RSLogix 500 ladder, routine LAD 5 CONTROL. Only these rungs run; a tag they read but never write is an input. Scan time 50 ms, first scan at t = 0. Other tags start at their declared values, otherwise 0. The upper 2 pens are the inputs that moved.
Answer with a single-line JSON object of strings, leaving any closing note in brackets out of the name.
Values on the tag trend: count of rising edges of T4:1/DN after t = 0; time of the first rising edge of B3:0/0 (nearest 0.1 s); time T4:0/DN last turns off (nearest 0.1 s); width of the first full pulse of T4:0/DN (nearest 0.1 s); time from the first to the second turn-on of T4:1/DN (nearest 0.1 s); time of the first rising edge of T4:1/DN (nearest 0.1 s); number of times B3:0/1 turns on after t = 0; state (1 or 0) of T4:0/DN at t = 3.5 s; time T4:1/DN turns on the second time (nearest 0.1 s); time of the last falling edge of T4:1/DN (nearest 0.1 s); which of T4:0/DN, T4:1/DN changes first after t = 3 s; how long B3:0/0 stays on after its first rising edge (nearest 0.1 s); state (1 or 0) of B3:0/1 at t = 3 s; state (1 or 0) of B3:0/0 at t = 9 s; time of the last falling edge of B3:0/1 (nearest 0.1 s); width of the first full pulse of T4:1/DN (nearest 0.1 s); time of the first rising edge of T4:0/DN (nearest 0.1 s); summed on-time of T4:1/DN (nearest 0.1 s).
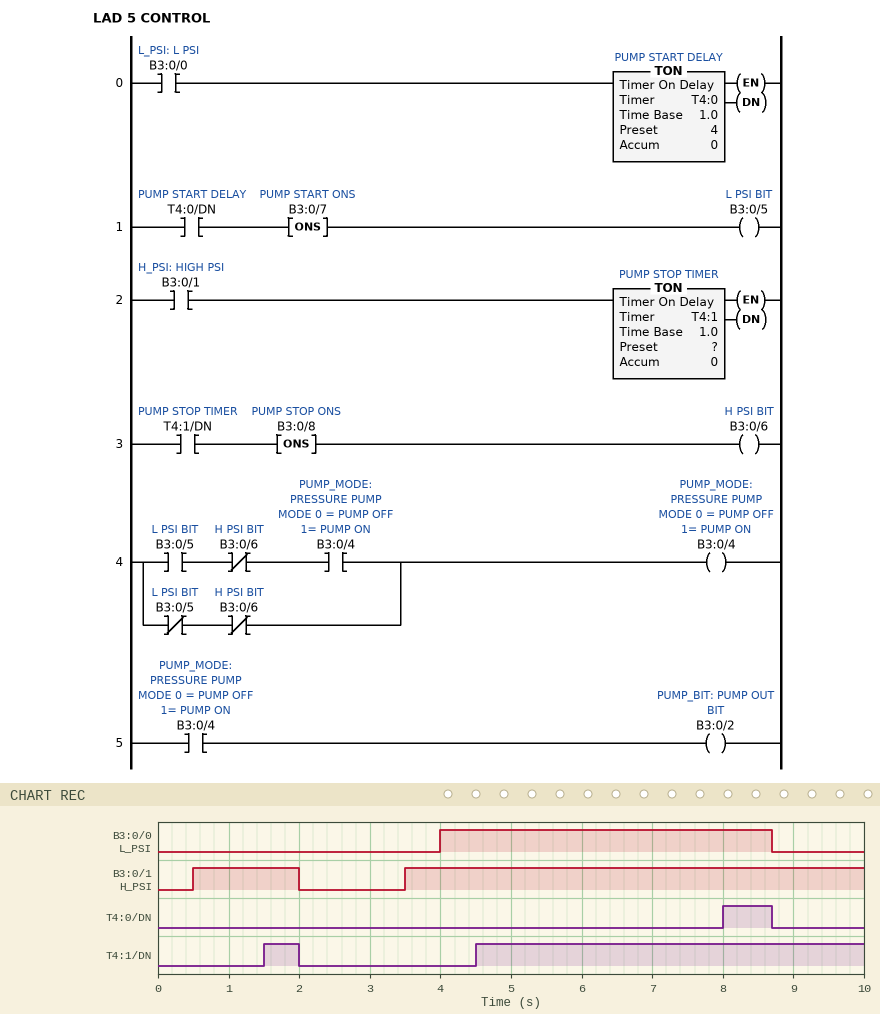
{"count of rising edges of T4:1/DN after t = 0": "2", "time of the first rising edge of B3:0/0": "4.0 s", "time T4:0/DN last turns off": "8.7 s", "width of the first full pulse of T4:0/DN": "0.7 s", "time from the first to the second turn-on of T4:1/DN": "3.0 s", "time of the first rising edge of T4:1/DN": "1.5 s", "number of times B3:0/1 turns on after t = 0": "2", "state (1 or 0) of T4:0/DN at t = 3.5 s": "0", "time T4:1/DN turns on the second time": "4.5 s", "time of the last falling edge of T4:1/DN": "2.0 s", "which of T4:0/DN, T4:1/DN changes first after t = 3 s": "T4:1/DN", "how long B3:0/0 stays on after its first rising edge": "4.7 s", "state (1 or 0) of B3:0/1 at t = 3 s": "0", "state (1 or 0) of B3:0/0 at t = 9 s": "0", "time of the last falling edge of B3:0/1": "2.0 s", "width of the first full pulse of T4:1/DN": "0.5 s", "time of the first rising edge of T4:0/DN": "8.0 s", "summed on-time of T4:1/DN": "6.0 s"}
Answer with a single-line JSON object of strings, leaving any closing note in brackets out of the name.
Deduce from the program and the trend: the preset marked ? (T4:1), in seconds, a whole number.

{"the preset marked ? (T4:1), in seconds, a whole number": "1 s"}
